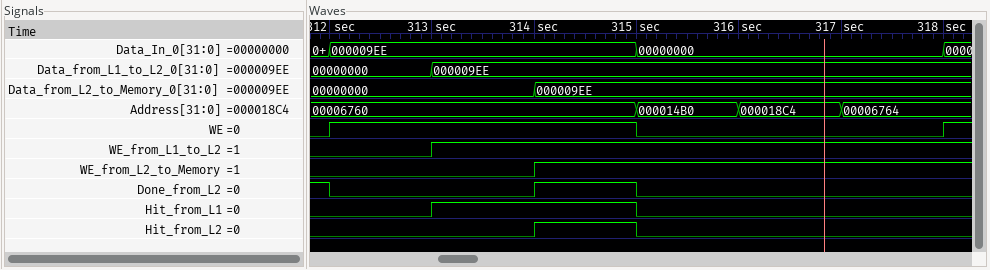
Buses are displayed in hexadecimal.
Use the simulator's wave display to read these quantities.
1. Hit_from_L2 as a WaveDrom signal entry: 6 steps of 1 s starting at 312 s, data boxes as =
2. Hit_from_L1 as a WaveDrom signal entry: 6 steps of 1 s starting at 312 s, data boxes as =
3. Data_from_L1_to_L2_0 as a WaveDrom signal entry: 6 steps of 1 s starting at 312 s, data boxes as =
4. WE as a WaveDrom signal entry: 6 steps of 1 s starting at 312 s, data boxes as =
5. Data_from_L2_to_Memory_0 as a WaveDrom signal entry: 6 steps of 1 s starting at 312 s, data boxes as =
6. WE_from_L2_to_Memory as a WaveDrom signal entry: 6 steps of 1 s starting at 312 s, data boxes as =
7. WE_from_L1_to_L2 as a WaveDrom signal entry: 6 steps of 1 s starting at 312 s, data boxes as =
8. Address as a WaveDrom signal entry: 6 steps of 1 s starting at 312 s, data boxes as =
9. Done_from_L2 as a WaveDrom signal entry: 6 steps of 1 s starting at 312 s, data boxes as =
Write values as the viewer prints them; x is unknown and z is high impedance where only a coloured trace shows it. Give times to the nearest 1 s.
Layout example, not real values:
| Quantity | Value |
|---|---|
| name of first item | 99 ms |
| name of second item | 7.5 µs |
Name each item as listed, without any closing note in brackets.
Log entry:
| Quantity | Value |
|---|---|
| Hit_from_L2 as a WaveDrom signal entry: 6 steps of 1 s starting at 312 s, data boxes as = | {name: 'Hit_from_L2', wave: '0.10..'} |
| Hit_from_L1 as a WaveDrom signal entry: 6 steps of 1 s starting at 312 s, data boxes as = | {name: 'Hit_from_L1', wave: '01.0..'} |
| Data_from_L1_to_L2_0 as a WaveDrom signal entry: 6 steps of 1 s starting at 312 s, data boxes as = | {name: 'Data_from_L1_to_L2_0', wave: '==....', data: '00000000 000009EE'} |
| WE as a WaveDrom signal entry: 6 steps of 1 s starting at 312 s, data boxes as = | {name: 'WE', wave: '1..0..'} |
| Data_from_L2_to_Memory_0 as a WaveDrom signal entry: 6 steps of 1 s starting at 312 s, data boxes as = | {name: 'Data_from_L2_to_Memory_0', wave: '=.=...', data: '00000000 000009EE'} |
| WE_from_L2_to_Memory as a WaveDrom signal entry: 6 steps of 1 s starting at 312 s, data boxes as = | {name: 'WE_from_L2_to_Memory', wave: '0.1...'} |
| WE_from_L1_to_L2 as a WaveDrom signal entry: 6 steps of 1 s starting at 312 s, data boxes as = | {name: 'WE_from_L1_to_L2', wave: '01....'} |
| Address as a WaveDrom signal entry: 6 steps of 1 s starting at 312 s, data boxes as = | {name: 'Address', wave: '=..===', data: '00006760 000014B0 000018C4 00006764'} |
| Done_from_L2 as a WaveDrom signal entry: 6 steps of 1 s starting at 312 s, data boxes as = | {name: 'Done_from_L2', wave: '0.10..'} |
